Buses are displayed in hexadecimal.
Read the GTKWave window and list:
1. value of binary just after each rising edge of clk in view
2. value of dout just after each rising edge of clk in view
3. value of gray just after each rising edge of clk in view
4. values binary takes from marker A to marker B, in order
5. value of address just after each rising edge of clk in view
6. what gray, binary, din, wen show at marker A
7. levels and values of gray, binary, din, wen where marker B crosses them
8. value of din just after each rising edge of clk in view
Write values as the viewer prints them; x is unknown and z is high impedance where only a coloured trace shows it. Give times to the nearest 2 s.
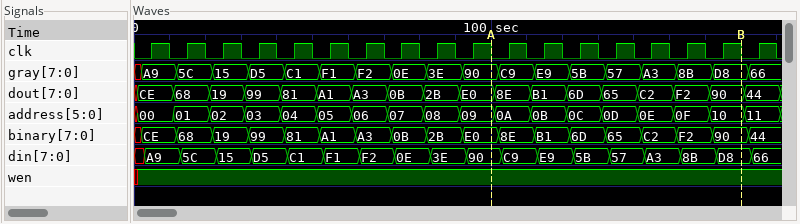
CE, 68, 19, 99, 81, A1, A3, 0B, 2B, E0, 8E, B1, 6D, 65, C2, F2, 90, 44
CE, 68, 19, 99, 81, A1, A3, 0B, 2B, E0, 8E, B1, 6D, 65, C2, F2, 90, 44
A9, 5C, 15, D5, C1, F1, F2, 0E, 3E, 90, C9, E9, 5B, 57, A3, 8B, D8, 66
E0, 8E, B1, 6D, 65, C2, F2, 90
00, 01, 02, 03, 04, 05, 06, 07, 08, 09, 0A, 0B, 0C, 0D, 0E, 0F, 10, 11
gray=90, binary=E0, din=90, wen=1
gray=D8, binary=90, din=D8, wen=1
A9, 5C, 15, D5, C1, F1, F2, 0E, 3E, 90, C9, E9, 5B, 57, A3, 8B, D8, 66
